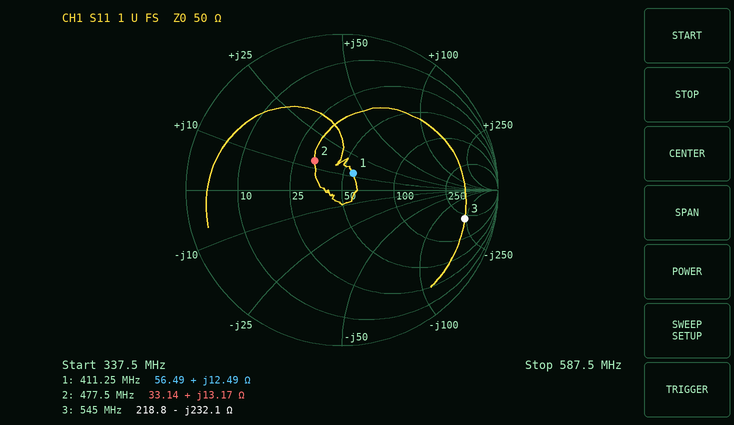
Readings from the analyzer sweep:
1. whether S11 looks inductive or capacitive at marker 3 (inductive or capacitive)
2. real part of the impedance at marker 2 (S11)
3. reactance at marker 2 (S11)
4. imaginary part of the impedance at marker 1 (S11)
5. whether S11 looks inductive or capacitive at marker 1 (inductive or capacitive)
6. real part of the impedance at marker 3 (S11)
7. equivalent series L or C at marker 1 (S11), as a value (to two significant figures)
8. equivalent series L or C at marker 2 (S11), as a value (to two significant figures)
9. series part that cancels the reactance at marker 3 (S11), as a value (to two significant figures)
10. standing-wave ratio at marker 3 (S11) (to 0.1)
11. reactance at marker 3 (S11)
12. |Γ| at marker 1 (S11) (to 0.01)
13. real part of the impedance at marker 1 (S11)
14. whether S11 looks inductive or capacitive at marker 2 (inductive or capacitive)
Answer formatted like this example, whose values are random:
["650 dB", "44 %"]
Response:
["capacitive", "33.14 Ω", "+13.17 Ω", "+12.49 Ω", "inductive", "218.8 Ω", "4.8 nH", "4.4 nH", "68 nH", "9.4", "-232.1 Ω", "0.13", "56.49 Ω", "inductive"]
